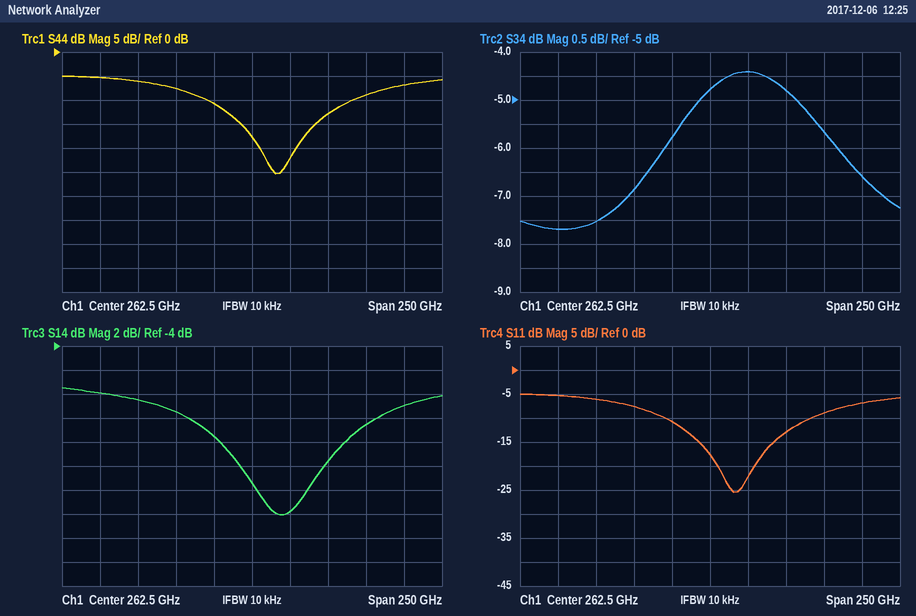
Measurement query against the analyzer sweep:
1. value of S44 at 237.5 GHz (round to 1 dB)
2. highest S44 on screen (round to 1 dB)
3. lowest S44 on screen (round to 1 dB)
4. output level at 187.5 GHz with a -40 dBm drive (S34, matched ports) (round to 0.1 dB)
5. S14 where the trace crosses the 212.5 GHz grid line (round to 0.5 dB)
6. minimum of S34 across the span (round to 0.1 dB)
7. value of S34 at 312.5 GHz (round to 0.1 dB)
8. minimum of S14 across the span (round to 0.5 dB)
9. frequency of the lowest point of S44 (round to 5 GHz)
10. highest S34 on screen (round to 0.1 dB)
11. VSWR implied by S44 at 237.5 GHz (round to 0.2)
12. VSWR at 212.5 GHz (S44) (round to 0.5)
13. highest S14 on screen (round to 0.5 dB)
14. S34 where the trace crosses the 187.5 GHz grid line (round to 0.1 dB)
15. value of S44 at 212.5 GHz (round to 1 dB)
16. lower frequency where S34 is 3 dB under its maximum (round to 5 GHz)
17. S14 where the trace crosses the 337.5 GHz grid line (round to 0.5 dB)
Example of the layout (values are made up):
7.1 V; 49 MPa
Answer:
-11 dB; -5 dB; -25 dB; -47.5 dBm; -9.5 dB; -7.7 dB; -4.8 dB; -18.0 dB; 280 GHz; -4.4 dB; 1.8; 2.5; -7.5 dB; -7.5 dB; -8 dB; 195 GHz; -10.5 dB
